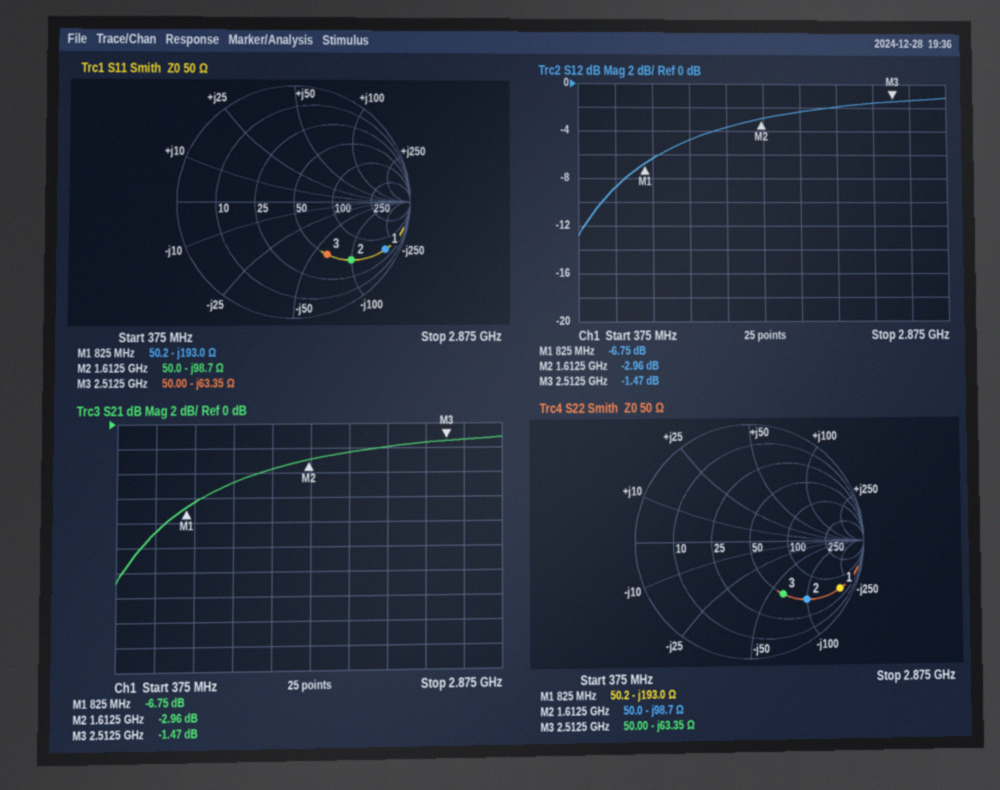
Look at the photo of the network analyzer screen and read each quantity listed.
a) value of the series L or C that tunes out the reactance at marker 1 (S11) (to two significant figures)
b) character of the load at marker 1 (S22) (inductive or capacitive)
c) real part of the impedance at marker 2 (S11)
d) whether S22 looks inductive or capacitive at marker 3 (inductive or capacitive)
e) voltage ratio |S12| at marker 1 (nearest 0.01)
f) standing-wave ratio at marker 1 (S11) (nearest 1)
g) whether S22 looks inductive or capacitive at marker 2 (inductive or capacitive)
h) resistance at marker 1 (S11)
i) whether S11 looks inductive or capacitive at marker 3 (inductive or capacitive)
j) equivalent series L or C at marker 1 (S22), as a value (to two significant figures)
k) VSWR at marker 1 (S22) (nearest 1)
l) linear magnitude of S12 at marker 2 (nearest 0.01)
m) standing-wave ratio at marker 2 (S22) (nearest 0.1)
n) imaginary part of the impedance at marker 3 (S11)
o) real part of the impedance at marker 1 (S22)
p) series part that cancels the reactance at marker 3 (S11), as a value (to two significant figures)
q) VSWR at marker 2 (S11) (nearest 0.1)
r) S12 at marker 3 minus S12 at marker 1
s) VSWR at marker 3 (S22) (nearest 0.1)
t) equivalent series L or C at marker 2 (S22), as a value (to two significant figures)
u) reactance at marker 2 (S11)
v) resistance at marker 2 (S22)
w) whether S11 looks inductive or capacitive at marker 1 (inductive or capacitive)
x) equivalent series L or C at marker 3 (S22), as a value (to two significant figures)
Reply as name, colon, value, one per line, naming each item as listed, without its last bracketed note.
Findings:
value of the series L or C that tunes out the reactance at marker 1 (S11): 37 nH
character of the load at marker 1 (S22): capacitive
real part of the impedance at marker 2: 50.0 Ω
whether S22 looks inductive or capacitive at marker 3: capacitive
voltage ratio |S12| at marker 1: 0.46
standing-wave ratio at marker 1 (S11): 17
whether S22 looks inductive or capacitive at marker 2: capacitive
resistance at marker 1: 50.2 Ω
whether S11 looks inductive or capacitive at marker 3: capacitive
equivalent series L or C at marker 1 (S22), as a value: 1.00 pF
VSWR at marker 1 (S22): 17
linear magnitude of S12 at marker 2: 0.71
standing-wave ratio at marker 2 (S22): 5.7
imaginary part of the impedance at marker 3: -63.35 Ω
real part of the impedance at marker 1: 50.2 Ω
series part that cancels the reactance at marker 3 (S11), as a value: 4.0 nH
VSWR at marker 2 (S11): 5.7
S12 at marker 3 minus S12 at marker 1: 5.28 dB
VSWR at marker 3 (S22): 3.3
equivalent series L or C at marker 2 (S22), as a value: 1.00 pF
reactance at marker 2: -98.7 Ω
resistance at marker 2: 50.0 Ω
whether S11 looks inductive or capacitive at marker 1: capacitive
equivalent series L or C at marker 3 (S22), as a value: 1.00 pF
